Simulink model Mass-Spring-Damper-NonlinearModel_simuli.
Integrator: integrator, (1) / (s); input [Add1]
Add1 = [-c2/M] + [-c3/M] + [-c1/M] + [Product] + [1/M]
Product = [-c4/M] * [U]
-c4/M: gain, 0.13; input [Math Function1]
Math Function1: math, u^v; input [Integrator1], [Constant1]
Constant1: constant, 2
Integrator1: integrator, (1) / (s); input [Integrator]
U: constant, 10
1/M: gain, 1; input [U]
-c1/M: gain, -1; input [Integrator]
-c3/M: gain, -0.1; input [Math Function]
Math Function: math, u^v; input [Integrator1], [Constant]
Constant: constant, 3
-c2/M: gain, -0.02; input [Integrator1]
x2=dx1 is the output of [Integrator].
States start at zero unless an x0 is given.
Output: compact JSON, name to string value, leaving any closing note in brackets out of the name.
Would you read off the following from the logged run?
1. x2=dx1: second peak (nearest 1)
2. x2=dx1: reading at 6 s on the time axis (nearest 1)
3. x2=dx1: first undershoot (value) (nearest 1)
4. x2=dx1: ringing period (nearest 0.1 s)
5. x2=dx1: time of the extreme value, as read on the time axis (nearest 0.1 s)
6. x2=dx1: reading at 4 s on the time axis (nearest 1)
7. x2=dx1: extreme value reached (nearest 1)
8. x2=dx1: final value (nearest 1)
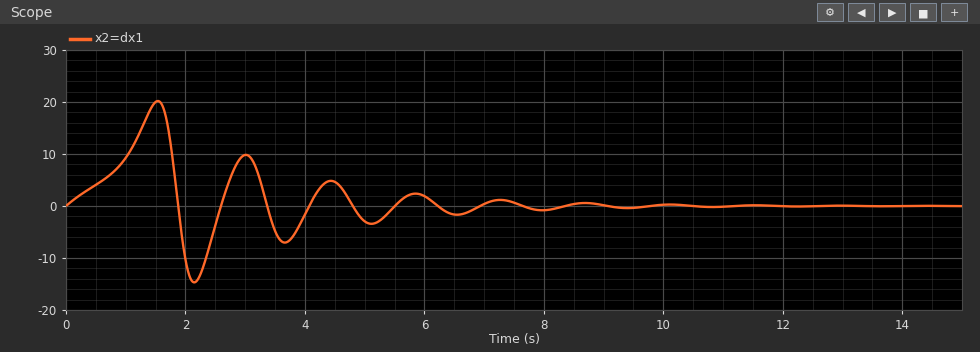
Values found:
{"x2=dx1: second peak": "10", "x2=dx1: reading at 6 s on the time axis": "2", "x2=dx1: first undershoot (value)": "-15", "x2=dx1: ringing period": "1.5 s", "x2=dx1: time of the extreme value, as read on the time axis": "1.5 s", "x2=dx1: reading at 4 s on the time axis": "-2", "x2=dx1: extreme value reached": "20", "x2=dx1: final value": "0"}
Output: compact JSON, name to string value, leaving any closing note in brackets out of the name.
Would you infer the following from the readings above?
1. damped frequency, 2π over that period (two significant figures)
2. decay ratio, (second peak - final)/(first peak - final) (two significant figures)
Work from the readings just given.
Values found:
{"damped frequency, 2π over that period": "4.2 rad/s", "decay ratio, (second peak - final)/(first peak - final)": "0.50"}
